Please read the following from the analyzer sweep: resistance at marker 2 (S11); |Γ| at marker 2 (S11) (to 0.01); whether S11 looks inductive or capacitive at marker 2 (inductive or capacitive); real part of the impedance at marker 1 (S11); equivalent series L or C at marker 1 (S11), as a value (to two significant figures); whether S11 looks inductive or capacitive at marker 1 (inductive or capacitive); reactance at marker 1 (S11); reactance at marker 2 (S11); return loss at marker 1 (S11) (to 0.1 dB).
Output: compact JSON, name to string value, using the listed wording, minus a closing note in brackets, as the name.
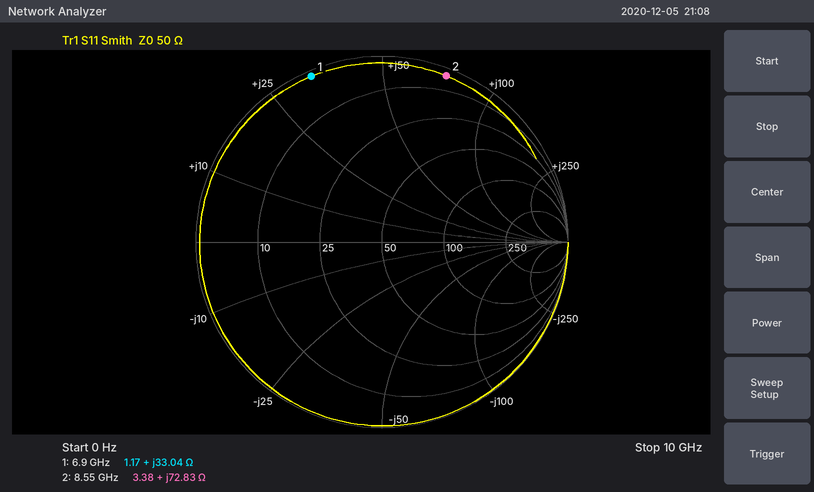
{"resistance at marker 2": "3.38 Ω", "|Γ| at marker 2 (S11)": "0.96", "whether S11 looks inductive or capacitive at marker 2": "inductive", "real part of the impedance at marker 1": "1.17 Ω", "equivalent series L or C at marker 1 (S11), as a value": "760 pH", "whether S11 looks inductive or capacitive at marker 1": "inductive", "reactance at marker 1": "+33.04 Ω", "reactance at marker 2": "+72.83 Ω", "return loss at marker 1 (S11)": "0.3 dB"}
